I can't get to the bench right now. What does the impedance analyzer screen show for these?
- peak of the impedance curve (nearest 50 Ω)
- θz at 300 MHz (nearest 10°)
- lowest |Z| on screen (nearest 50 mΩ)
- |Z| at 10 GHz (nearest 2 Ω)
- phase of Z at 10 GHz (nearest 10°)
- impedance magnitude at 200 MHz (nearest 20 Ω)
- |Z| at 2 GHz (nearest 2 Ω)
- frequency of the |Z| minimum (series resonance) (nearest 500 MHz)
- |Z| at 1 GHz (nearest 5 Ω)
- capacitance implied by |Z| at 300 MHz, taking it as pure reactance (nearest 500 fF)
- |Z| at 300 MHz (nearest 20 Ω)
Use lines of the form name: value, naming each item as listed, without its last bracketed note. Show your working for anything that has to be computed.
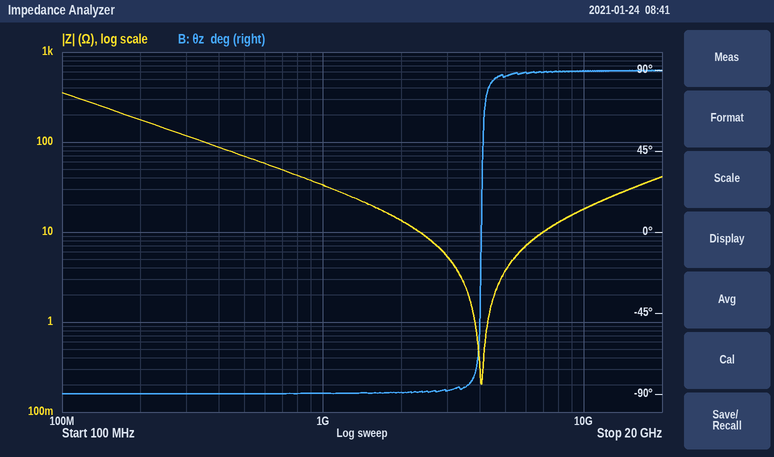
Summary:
peak of the impedance curve: 350 Ω
θz at 300 MHz: -90°
lowest |Z| on screen: 200 mΩ
|Z| at 10 GHz: 18 Ω
phase of Z at 10 GHz: 90°
impedance magnitude at 200 MHz: 180 Ω
|Z| at 2 GHz: 14 Ω
frequency of the |Z| minimum (series resonance): 4.0 GHz
|Z| at 1 GHz: 35 Ω
capacitance implied by |Z| at 300 MHz, taking it as pure reactance: C = 1/(2π × 300 MHz × 120 Ω) ≈ 4.42 pF, so 4.5 pF to the nearest 500 fF
|Z| at 300 MHz: 120 Ω
